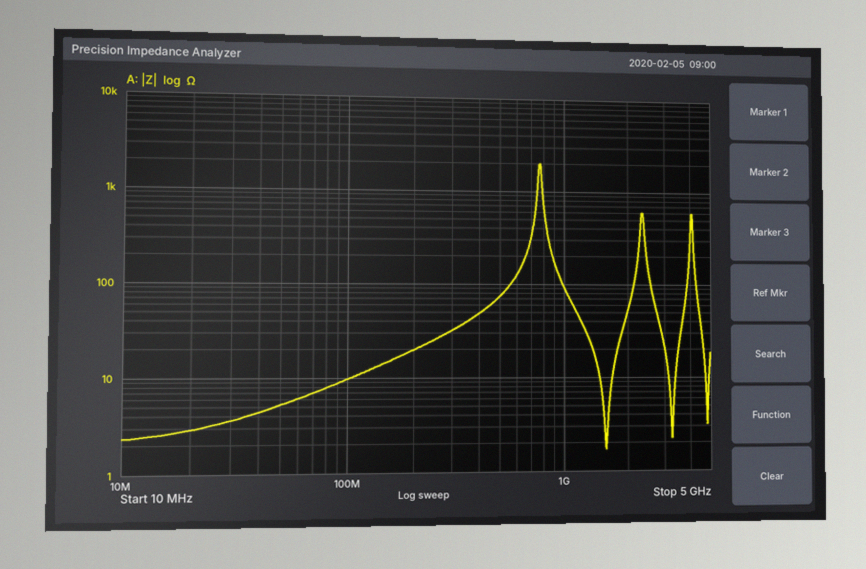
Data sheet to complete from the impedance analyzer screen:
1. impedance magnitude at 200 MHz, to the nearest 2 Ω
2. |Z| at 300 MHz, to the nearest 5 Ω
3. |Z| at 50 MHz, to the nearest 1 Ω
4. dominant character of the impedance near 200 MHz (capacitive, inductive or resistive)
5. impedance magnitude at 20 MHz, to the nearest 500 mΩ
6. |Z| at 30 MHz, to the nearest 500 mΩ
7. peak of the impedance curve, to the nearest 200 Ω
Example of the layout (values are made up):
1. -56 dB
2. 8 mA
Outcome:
1. 20 Ω
2. 30 Ω
3. 5 Ω
4. inductive
5. 3.0 Ω
6. 3.5 Ω
7. 2.0 kΩ
